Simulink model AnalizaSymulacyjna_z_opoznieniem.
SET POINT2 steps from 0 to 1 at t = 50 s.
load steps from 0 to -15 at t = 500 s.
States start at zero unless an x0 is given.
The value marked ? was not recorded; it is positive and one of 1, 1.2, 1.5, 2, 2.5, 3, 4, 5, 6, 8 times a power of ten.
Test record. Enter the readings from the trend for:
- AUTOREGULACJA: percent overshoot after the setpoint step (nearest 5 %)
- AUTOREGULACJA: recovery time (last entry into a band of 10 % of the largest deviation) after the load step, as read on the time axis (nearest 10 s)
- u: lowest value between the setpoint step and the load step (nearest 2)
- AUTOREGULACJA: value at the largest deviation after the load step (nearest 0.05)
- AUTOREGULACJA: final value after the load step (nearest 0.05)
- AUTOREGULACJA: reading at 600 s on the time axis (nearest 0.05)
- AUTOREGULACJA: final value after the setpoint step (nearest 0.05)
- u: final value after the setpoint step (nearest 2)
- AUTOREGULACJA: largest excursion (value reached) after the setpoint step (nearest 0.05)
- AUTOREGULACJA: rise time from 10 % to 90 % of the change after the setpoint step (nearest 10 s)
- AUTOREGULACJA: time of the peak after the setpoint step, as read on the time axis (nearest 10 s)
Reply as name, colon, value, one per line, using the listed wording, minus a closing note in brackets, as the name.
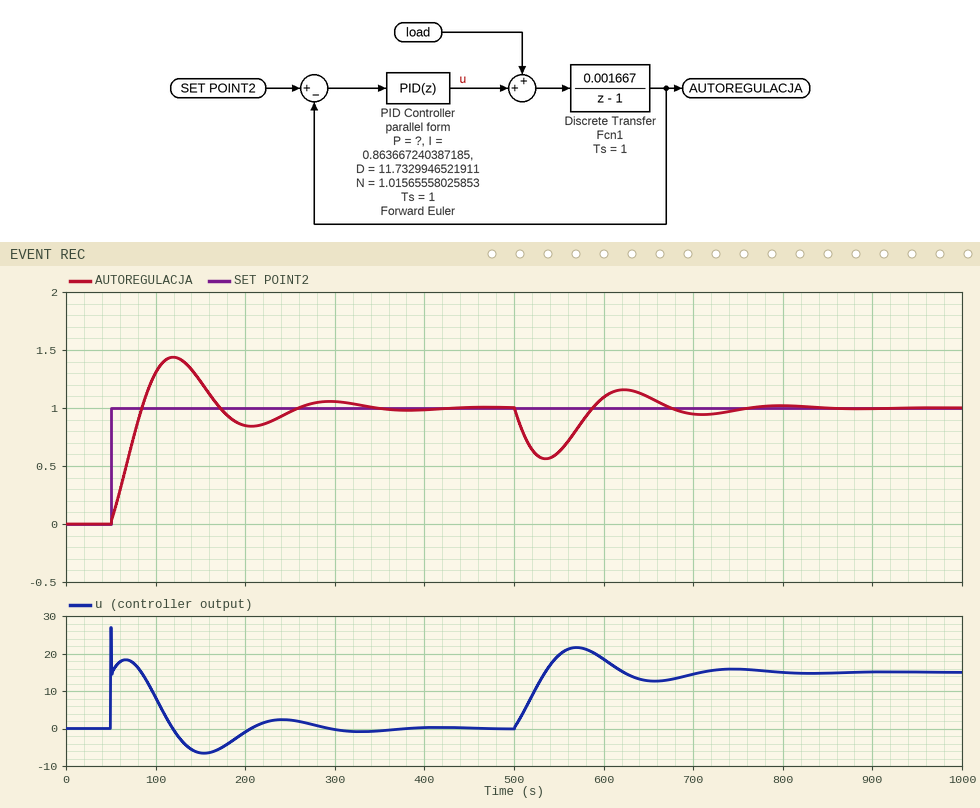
AUTOREGULACJA: percent overshoot after the setpoint step: 45 %
AUTOREGULACJA: recovery time (last entry into a band of 10 % of the largest deviation) after the load step, as read on the time axis: 730 s
u: lowest value between the setpoint step and the load step: -6
AUTOREGULACJA: value at the largest deviation after the load step: 0.55
AUTOREGULACJA: final value after the load step: 1.00
AUTOREGULACJA: reading at 600 s on the time axis: 1.10
AUTOREGULACJA: final value after the setpoint step: 1.00
u: final value after the setpoint step: 0
AUTOREGULACJA: largest excursion (value reached) after the setpoint step: 1.45
AUTOREGULACJA: rise time from 10 % to 90 % of the change after the setpoint step: 30 s
AUTOREGULACJA: time of the peak after the setpoint step, as read on the time axis: 120 s
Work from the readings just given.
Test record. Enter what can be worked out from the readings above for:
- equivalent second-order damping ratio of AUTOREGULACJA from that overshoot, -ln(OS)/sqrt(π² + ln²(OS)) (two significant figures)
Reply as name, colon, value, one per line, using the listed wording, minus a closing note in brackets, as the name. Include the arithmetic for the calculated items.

equivalent second-order damping ratio of AUTOREGULACJA from that overshoot, -ln(OS)/sqrt(π² + ln²(OS)): ln(0.45) = -0.799; 0.799 / sqrt(9.870 + 0.638) = 0.25
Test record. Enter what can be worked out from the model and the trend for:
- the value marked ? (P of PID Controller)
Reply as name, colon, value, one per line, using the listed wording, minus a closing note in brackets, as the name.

the value marked ?: 15
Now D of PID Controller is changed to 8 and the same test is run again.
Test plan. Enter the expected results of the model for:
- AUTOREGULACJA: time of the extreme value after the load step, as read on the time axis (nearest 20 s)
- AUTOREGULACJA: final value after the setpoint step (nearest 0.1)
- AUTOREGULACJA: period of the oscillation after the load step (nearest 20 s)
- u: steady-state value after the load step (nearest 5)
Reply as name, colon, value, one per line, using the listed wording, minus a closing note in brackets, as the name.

AUTOREGULACJA: time of the extreme value after the load step, as read on the time axis: 540 s
AUTOREGULACJA: final value after the setpoint step: 1.0
AUTOREGULACJA: period of the oscillation after the load step: 180 s
u: steady-state value after the load step: 15
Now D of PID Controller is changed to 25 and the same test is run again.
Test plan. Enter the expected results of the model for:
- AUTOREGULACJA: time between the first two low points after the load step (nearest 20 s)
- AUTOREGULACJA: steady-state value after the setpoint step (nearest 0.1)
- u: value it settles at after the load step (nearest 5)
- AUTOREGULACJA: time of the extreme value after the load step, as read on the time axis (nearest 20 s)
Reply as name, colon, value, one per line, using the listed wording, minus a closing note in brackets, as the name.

AUTOREGULACJA: time between the first two low points after the load step: 180 s
AUTOREGULACJA: steady-state value after the setpoint step: 1.0
u: value it settles at after the load step: 15
AUTOREGULACJA: time of the extreme value after the load step, as read on the time axis: 540 s
